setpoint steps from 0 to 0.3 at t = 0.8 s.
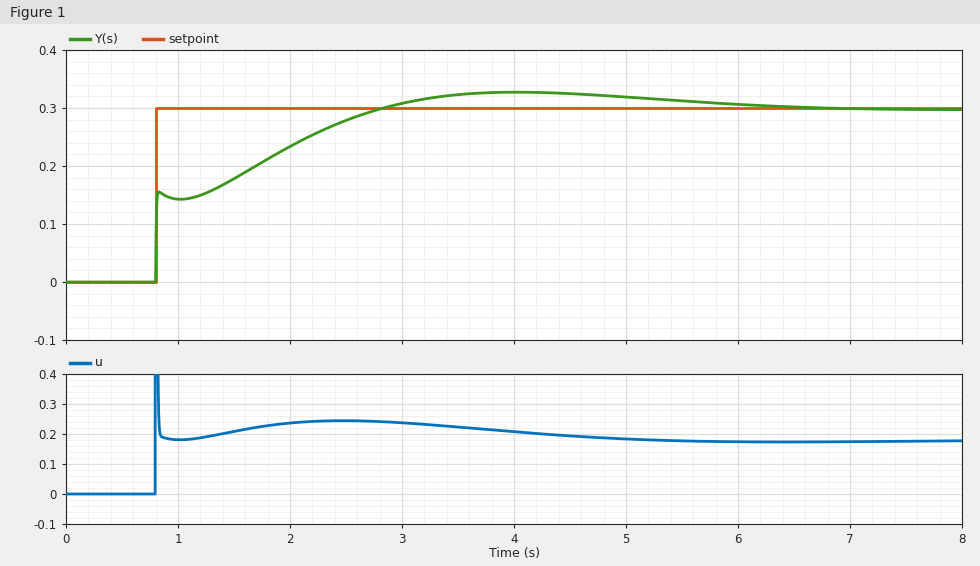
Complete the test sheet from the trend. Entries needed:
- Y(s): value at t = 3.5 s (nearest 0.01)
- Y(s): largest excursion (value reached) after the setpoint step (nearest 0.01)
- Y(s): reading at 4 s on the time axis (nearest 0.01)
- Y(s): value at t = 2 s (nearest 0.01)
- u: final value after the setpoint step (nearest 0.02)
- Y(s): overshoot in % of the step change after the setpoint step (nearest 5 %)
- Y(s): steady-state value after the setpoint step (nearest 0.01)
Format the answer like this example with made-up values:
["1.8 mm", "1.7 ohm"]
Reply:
["0.32", "0.33", "0.33", "0.23", "0.18", "10 %", "0.30"]
